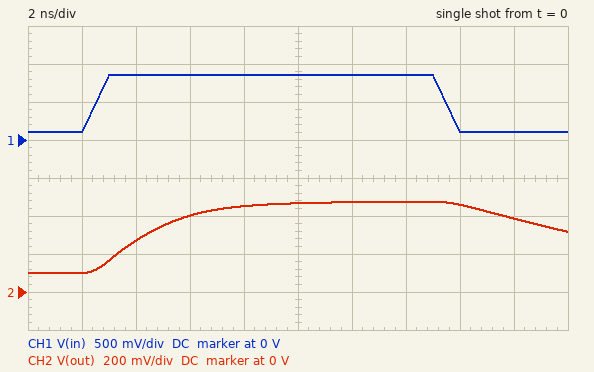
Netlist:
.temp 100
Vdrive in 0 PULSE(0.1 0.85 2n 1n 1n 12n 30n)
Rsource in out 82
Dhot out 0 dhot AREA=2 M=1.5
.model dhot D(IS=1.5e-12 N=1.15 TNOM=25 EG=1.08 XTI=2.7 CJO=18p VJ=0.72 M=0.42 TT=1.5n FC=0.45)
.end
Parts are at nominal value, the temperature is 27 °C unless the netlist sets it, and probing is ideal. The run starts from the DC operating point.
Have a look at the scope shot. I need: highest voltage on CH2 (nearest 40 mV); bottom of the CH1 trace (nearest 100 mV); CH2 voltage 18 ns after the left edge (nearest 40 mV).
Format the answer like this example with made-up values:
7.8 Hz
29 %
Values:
480 mV
100 mV
400 mV
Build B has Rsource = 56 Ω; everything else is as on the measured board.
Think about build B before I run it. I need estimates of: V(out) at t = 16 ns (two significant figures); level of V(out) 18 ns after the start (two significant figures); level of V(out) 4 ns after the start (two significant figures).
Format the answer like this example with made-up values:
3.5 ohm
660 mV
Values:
470 mV
370 mV
330 mV
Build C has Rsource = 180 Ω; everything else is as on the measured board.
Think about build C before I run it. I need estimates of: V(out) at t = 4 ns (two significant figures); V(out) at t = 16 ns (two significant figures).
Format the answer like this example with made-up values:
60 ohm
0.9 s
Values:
190 mV
430 mV
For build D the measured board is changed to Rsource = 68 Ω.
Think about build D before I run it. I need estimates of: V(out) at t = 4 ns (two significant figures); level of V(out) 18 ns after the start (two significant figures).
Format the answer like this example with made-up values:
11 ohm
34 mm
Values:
300 mV
380 mV
